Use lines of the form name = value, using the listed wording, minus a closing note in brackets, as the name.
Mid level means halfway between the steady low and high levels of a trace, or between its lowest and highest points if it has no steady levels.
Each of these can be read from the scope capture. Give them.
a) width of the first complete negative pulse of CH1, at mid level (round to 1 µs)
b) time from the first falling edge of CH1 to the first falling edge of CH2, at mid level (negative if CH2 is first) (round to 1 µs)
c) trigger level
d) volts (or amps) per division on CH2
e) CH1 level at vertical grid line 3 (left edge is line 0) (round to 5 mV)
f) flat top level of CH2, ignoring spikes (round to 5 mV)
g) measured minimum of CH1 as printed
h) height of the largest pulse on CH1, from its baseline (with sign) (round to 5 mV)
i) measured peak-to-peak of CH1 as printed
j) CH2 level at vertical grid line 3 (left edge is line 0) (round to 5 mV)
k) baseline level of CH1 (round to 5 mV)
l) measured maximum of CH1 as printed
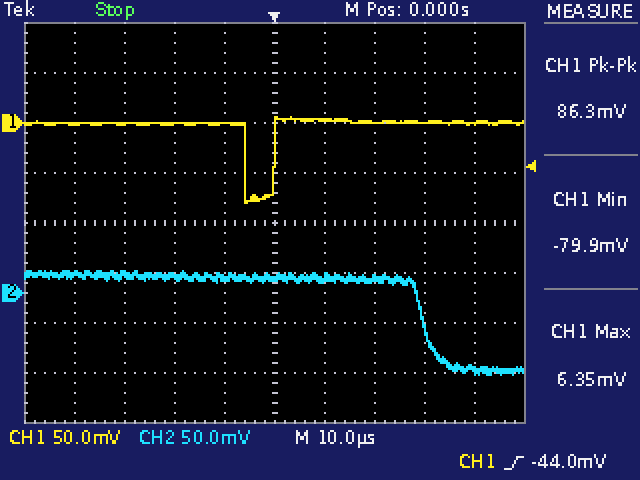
width of the first complete negative pulse of CH1, at mid level = 6 µs
time from the first falling edge of CH1 to the first falling edge of CH2, at mid level (negative if CH2 is first) = +36 µs
trigger level = -44.0 mV
volts (or amps) per division on CH2 = 50 mV
CH1 level at vertical grid line 3 (left edge is line 0) = 0 mV
flat top level of CH2, ignoring spikes = 15 mV
measured minimum of CH1 as printed = -79.9 mV
height of the largest pulse on CH1, from its baseline (with sign) = -80 mV
measured peak-to-peak of CH1 as printed = 86.3 mV
CH2 level at vertical grid line 3 (left edge is line 0) = 15 mV
baseline level of CH1 = 0 mV
measured maximum of CH1 as printed = 6.35 mV
